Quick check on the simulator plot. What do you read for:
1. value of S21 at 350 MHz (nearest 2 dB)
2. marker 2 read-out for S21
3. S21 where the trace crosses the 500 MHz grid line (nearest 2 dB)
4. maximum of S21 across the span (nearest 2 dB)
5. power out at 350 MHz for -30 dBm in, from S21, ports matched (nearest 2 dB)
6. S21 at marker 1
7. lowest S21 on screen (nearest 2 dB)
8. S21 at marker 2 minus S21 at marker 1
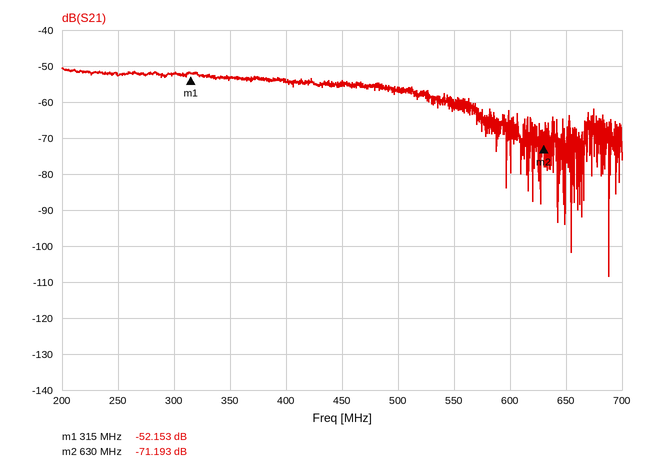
-54 dB
-71.193 dB
-56 dB
-50 dB
-84 dBm
-52.153 dB
-108 dB
-19.040 dB
